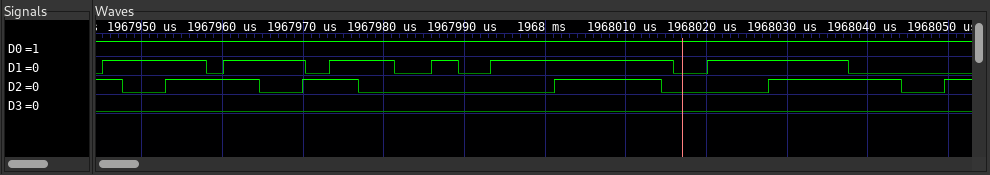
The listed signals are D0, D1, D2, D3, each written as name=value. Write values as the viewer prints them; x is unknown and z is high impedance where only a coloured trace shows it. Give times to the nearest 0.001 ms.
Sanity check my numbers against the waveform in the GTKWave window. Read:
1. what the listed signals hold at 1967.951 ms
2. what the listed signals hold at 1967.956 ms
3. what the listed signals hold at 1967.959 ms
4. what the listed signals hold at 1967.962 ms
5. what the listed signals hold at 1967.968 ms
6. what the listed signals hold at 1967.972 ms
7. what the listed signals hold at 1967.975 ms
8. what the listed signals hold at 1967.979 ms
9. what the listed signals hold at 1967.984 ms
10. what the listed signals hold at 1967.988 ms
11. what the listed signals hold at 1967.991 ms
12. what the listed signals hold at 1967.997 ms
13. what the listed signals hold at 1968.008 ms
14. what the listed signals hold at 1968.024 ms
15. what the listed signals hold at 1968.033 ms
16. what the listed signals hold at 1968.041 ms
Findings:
D0=1, D1=1, D2=0, D3=0
D0=1, D1=1, D2=1, D3=0
D0=1, D1=0, D2=1, D3=0
D0=1, D1=1, D2=1, D3=0
D0=1, D1=1, D2=0, D3=0
D0=1, D1=0, D2=1, D3=0
D0=1, D1=1, D2=1, D3=0
D0=1, D1=1, D2=0, D3=0
D0=1, D1=0, D2=0, D3=0
D0=1, D1=1, D2=0, D3=0
D0=1, D1=0, D2=0, D3=0
D0=1, D1=1, D2=0, D3=0
D0=1, D1=1, D2=1, D3=0
D0=1, D1=1, D2=0, D3=0
D0=1, D1=1, D2=1, D3=0
D0=1, D1=0, D2=1, D3=0
